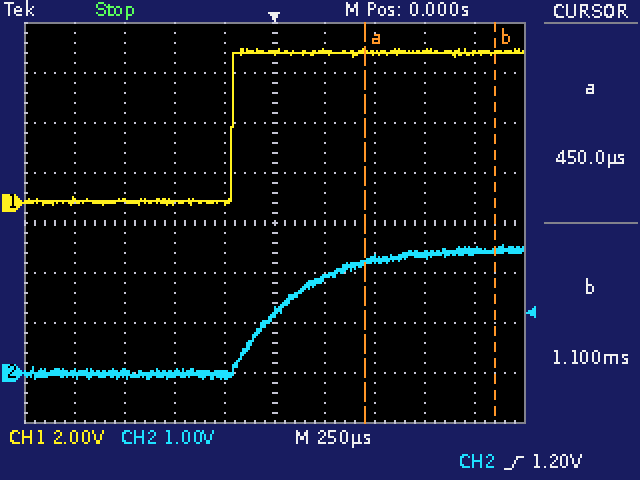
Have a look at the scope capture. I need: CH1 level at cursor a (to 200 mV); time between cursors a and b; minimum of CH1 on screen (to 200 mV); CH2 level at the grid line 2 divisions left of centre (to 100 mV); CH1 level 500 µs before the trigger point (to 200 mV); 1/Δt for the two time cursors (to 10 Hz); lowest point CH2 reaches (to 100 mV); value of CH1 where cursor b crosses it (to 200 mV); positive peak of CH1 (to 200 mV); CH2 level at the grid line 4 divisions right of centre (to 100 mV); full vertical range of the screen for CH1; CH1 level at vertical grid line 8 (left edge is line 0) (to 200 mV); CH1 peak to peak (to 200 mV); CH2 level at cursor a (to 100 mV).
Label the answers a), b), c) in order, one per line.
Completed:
a) 6.0 V
b) 650 µs
c) 0.0 V
d) 0.0 V
e) 0.0 V
f) 1.54 kHz
g) -100 mV
h) 6.0 V
i) 6.2 V
j) 2.4 V
k) 16 V
l) 6.0 V
m) 6.2 V
n) 2.2 V
